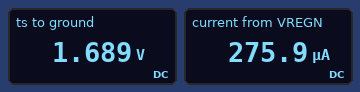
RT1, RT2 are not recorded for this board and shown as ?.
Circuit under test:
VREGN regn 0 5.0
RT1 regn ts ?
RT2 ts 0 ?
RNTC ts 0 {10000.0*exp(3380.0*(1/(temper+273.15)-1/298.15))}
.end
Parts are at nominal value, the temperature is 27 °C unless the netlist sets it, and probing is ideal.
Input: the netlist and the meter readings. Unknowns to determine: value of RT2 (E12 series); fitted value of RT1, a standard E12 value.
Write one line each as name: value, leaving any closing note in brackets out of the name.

value of RT2: 18 kΩ
fitted value of RT1, a standard E12 value: 12 kΩ
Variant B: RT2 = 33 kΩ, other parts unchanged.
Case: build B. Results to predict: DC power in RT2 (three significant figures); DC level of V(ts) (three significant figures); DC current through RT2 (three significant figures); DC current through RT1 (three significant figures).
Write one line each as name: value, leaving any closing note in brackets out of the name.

DC power in RT2: 107 µW
DC level of V(ts): 1.88 V
DC current through RT2: 57.0 µA
DC current through RT1: 260 µA
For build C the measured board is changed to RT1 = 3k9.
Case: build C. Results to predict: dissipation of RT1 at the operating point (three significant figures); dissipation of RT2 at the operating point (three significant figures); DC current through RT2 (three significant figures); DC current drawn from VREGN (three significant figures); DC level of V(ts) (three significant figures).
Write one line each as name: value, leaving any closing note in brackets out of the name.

dissipation of RT1 at the operating point: 971 µW
dissipation of RT2 at the operating point: 518 µW
DC current through RT2: 170 µA
DC current drawn from VREGN: 499 µA
DC level of V(ts): 3.05 V
